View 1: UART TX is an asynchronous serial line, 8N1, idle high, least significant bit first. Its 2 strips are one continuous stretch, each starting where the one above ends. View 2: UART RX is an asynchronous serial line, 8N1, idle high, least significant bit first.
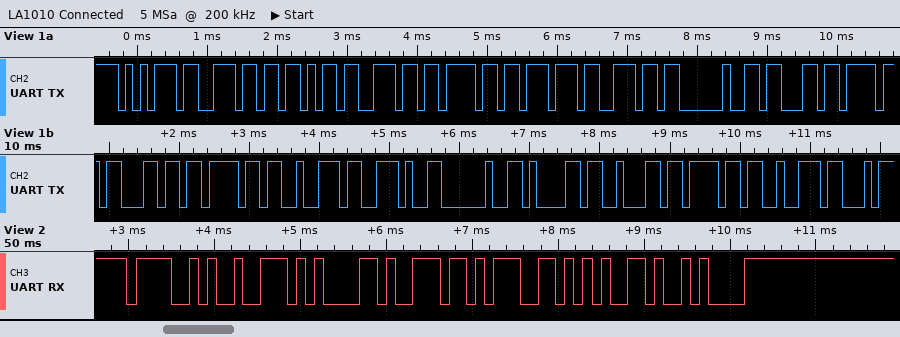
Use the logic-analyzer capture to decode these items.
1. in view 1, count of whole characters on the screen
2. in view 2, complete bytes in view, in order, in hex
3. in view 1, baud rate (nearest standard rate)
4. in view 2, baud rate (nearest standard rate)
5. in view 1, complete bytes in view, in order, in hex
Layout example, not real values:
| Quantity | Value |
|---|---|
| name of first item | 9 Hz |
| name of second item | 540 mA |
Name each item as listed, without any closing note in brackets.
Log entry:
| Quantity | Value |
|---|---|
| in view 1, count of whole characters on the screen | 19 |
| in view 2, complete bytes in view, in order, in hex | 0x4F 0x72 0x61 0x6E 0x67 0x65 0x0A |
| in view 1, baud rate | 9600 baud |
| in view 2, baud rate | 9600 baud |
| in view 1, complete bytes in view, in order, in hex | 75 6E 6B 6E 6F 77 6E 20 63 6F 6C 6F 72 2E 20 61 62 6F 72 |
